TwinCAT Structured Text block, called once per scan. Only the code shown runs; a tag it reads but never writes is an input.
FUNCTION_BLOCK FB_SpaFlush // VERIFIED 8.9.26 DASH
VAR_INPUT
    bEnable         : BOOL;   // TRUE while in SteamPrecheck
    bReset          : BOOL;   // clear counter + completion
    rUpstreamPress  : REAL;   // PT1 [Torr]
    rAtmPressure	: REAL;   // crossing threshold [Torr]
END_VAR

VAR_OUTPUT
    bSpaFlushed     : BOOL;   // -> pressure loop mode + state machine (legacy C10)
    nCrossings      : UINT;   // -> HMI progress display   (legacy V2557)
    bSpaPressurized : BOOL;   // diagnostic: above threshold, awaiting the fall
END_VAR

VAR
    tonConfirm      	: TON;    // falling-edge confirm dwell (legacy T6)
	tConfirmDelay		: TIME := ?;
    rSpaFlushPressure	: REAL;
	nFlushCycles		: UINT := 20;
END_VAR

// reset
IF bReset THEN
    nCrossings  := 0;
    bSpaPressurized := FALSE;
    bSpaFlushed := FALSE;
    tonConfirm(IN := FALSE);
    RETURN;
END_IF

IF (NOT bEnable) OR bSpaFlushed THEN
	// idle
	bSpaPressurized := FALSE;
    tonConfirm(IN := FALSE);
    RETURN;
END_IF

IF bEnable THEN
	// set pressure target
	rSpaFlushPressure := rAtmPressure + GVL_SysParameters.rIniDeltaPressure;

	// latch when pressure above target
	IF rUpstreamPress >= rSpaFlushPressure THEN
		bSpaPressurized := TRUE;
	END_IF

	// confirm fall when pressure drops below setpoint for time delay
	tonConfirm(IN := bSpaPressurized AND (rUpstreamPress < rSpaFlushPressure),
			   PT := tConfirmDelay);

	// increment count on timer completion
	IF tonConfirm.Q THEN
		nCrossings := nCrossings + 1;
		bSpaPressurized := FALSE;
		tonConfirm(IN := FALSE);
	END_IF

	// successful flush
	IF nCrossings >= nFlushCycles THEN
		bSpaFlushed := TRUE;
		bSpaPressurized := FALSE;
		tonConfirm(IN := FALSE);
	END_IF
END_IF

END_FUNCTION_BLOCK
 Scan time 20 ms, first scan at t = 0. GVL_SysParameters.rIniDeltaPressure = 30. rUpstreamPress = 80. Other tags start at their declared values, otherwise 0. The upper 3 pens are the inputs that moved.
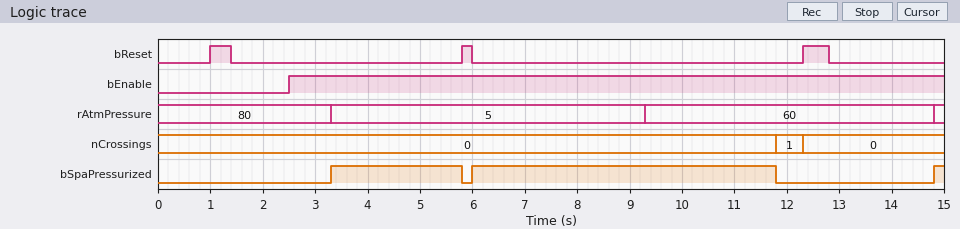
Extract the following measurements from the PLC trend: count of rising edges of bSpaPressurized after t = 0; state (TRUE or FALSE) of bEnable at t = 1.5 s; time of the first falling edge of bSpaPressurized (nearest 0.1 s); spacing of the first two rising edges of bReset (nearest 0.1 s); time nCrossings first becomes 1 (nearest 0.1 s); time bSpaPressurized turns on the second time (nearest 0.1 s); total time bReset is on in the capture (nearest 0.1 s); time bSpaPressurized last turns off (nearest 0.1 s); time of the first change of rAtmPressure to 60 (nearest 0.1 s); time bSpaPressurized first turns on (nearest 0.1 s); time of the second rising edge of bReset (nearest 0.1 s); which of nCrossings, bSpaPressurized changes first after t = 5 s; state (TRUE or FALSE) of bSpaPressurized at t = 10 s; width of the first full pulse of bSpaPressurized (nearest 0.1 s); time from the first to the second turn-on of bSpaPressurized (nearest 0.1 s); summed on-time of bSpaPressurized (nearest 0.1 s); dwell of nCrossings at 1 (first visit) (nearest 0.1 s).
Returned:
3
FALSE
5.8 s
4.8 s
11.8 s
6.0 s
1.1 s
11.8 s
9.3 s
3.3 s
5.8 s
bSpaPressurized
TRUE
2.5 s
2.7 s
8.5 s
0.5 s
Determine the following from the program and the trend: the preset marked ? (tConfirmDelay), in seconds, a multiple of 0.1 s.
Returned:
2.5 s
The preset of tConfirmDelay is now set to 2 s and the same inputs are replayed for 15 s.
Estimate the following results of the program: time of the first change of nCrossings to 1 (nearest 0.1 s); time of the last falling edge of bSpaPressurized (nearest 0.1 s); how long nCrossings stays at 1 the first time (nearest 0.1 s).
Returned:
11.3 s
11.3 s
1.0 s
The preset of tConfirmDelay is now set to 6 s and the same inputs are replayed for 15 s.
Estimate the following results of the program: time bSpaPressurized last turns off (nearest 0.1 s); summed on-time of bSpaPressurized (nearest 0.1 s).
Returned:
12.3 s
9.0 s
